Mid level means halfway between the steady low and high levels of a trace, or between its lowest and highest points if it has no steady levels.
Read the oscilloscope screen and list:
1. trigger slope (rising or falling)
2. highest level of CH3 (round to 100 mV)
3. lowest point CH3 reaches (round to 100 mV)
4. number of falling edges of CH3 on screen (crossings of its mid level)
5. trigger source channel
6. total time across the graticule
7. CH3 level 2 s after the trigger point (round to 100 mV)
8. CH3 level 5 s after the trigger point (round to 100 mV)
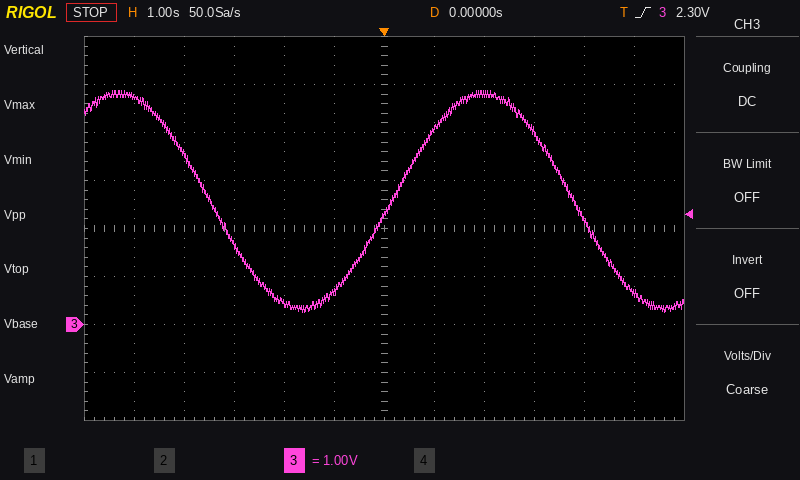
rising
4.9 V
200 mV
2
CH3
12 s
4.8 V
700 mV
